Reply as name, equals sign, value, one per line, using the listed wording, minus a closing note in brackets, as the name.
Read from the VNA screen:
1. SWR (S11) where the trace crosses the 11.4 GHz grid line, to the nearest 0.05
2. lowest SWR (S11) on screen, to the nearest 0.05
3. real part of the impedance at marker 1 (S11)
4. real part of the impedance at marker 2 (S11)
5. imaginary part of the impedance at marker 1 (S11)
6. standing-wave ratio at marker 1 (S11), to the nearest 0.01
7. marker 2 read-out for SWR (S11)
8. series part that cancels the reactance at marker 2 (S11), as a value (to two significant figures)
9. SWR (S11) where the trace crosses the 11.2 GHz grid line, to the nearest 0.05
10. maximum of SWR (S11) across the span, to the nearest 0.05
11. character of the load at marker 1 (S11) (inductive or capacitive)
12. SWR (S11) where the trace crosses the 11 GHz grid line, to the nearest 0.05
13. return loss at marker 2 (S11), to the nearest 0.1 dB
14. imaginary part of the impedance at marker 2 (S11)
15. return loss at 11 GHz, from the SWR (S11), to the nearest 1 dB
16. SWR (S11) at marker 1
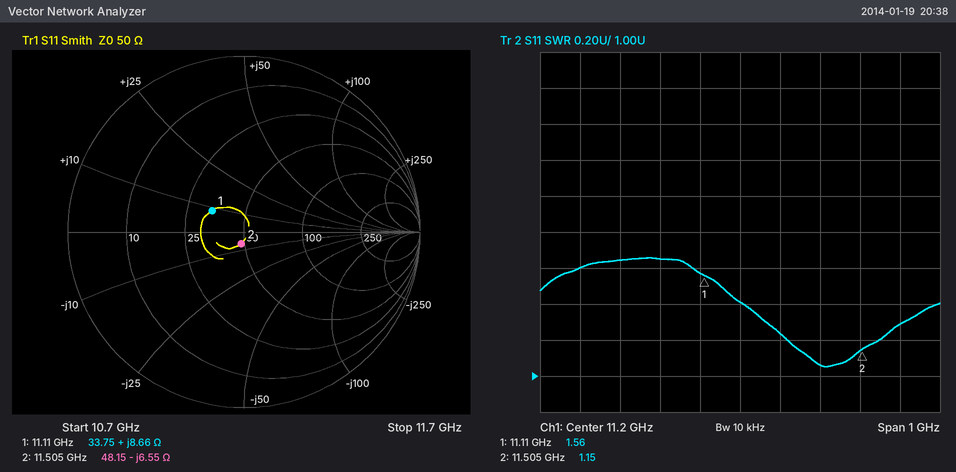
SWR (S11) where the trace crosses the 11.4 GHz grid line, to the nearest 0.05 = 1.05
lowest SWR (S11) on screen, to the nearest 0.05 = 1.05
real part of the impedance at marker 1 = 33.75 Ω
real part of the impedance at marker 2 = 48.15 Ω
imaginary part of the impedance at marker 1 = +8.66 Ω
standing-wave ratio at marker 1 (S11), to the nearest 0.01 = 1.56
marker 2 read-out for SWR = 1.15
series part that cancels the reactance at marker 2 (S11), as a value = 91 pH
SWR (S11) where the trace crosses the 11.2 GHz grid line, to the nearest 0.05 = 1.40
maximum of SWR (S11) across the span, to the nearest 0.05 = 1.65
character of the load at marker 1 (S11) = inductive
SWR (S11) where the trace crosses the 11 GHz grid line, to the nearest 0.05 = 1.65
return loss at marker 2 (S11), to the nearest 0.1 dB = 23.2 dB
imaginary part of the impedance at marker 2 = -6.55 Ω
return loss at 11 GHz, from the SWR (S11), to the nearest 1 dB = 12 dB
SWR (S11) at marker 1 = 1.56
